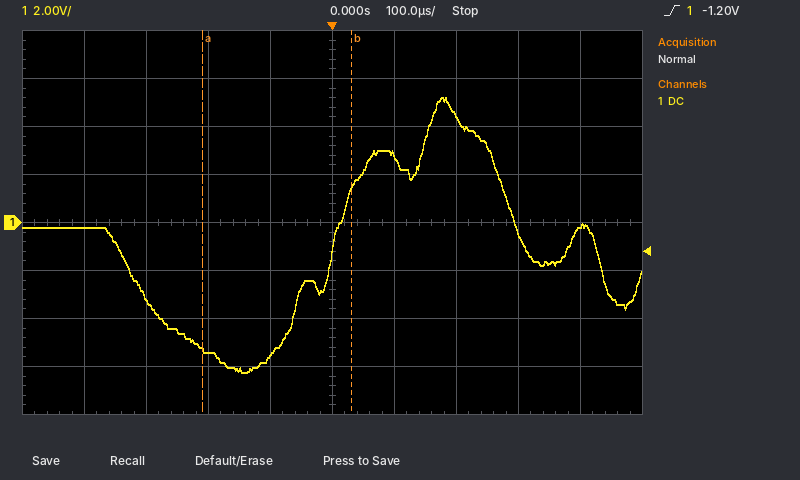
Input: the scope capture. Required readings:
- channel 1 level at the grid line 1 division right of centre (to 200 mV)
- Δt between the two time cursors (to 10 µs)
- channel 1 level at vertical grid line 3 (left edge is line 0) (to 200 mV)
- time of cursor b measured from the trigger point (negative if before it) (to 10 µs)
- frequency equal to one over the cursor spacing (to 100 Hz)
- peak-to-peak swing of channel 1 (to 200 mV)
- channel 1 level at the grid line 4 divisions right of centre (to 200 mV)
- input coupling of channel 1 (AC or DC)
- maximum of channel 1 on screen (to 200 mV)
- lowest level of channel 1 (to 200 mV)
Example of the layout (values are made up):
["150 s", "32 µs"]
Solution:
["2.8 V", "240 µs", "-5.4 V", "+30 µs", "4.2 kHz", "11.4 V", "-200 mV", "DC", "5.2 V", "-6.2 V"]
